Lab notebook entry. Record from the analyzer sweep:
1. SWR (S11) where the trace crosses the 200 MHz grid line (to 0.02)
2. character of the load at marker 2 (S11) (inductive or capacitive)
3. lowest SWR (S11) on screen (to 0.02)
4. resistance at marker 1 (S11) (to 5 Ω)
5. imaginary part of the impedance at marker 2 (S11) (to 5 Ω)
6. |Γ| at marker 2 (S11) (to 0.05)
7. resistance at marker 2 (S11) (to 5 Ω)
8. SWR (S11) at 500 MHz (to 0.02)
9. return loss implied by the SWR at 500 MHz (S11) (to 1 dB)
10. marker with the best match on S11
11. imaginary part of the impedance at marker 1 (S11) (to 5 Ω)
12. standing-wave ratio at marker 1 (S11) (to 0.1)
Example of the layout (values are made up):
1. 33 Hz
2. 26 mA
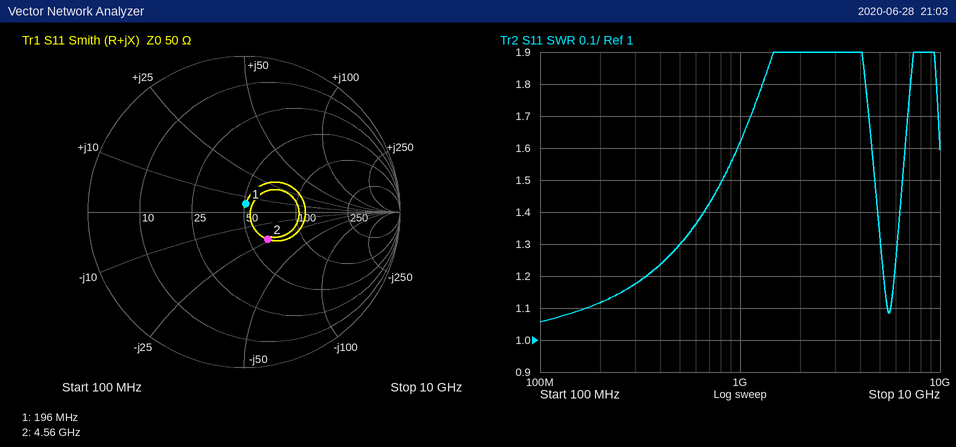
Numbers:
1. 1.12
2. capacitive
3. 1.06
4. 50 Ω
5. -25 Ω
6. 0.25
7. 65 Ω
8. 1.30
9. 18 dB
10. marker 1
11. +5 Ω
12. 1.1
